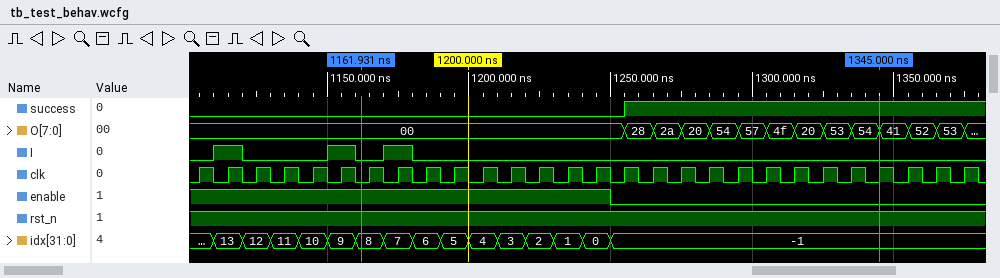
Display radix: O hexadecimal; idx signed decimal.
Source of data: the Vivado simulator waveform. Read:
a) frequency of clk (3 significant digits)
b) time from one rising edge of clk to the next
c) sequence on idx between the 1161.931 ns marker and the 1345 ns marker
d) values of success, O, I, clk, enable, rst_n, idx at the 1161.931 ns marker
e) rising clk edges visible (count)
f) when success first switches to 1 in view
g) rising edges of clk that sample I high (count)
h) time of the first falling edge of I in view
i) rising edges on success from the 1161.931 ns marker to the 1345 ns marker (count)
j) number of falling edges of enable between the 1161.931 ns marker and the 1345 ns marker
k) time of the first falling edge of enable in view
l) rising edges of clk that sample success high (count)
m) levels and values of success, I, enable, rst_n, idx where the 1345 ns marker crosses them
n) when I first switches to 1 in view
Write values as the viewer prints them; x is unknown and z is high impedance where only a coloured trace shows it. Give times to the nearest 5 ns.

100 MHz
10 ns
8, 7, 6, 5, 4, 3, 2, 1, 0, -1
success=0, O=00, I=0, clk=0, enable=1, rst_n=1, idx=8
28
1255 ns
3
1120 ns
1
1
1250 ns
12
success=1, I=0, enable=0, rst_n=1, idx=-1
1110 ns
